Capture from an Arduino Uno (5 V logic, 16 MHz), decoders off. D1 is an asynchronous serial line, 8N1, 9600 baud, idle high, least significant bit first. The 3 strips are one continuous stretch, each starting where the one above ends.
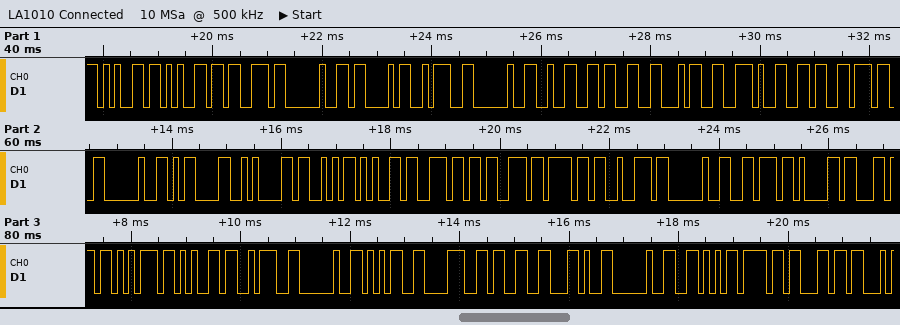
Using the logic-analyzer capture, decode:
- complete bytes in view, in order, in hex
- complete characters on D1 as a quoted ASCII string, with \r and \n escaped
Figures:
65 65 73 20 43 3A 20 32 33 34 2E 36 37 20 0D 0A 53 65 6E 73 6F 72 20 76 61 6C 75 65 3A 20 35 38 33 2C 20 56 6F 6C
"ees C: 234.67 \r\nSensor value: 583, Vol"
